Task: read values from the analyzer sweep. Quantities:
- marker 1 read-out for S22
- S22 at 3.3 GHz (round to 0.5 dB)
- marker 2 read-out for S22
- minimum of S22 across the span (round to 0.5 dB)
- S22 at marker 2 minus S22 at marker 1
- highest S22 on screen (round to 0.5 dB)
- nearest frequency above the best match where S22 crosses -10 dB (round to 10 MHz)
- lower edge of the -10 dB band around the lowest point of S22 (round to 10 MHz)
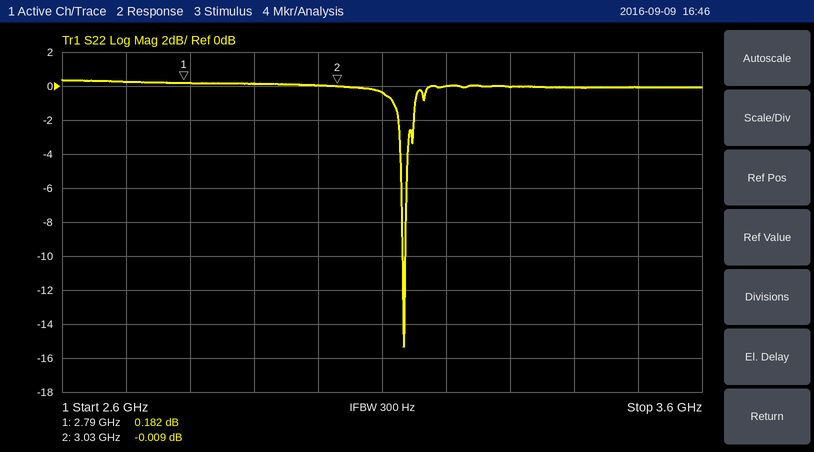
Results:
0.182 dB
0.0 dB
-0.009 dB
-15.5 dB
-0.191 dB
0.5 dB
3.14 GHz
3.13 GHz
